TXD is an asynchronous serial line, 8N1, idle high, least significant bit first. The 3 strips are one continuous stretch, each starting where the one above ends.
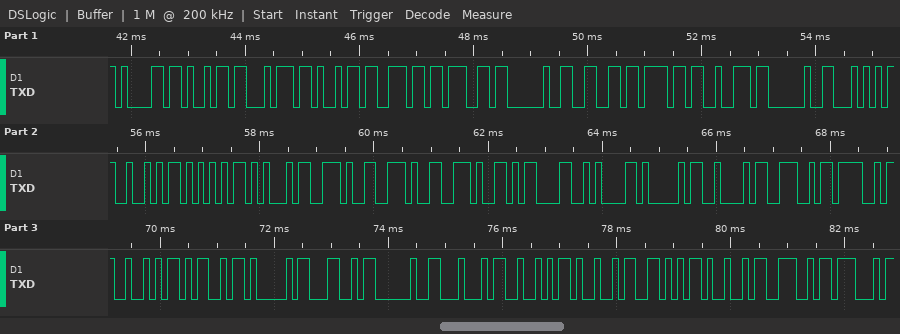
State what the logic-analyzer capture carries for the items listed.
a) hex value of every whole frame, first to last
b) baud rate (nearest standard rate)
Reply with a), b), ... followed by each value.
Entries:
a) 0x61 0x69 0x74 0x69 0x6E 0x67 0x20 0x66 0x6F 0x72 0x20 0x54 0x52 0x55 0x45 0x2E 0x2E 0x2E 0x0D 0x0A 0x41 0x42 0x4E 0x4F 0x52 0x4D 0x41 0x4C 0x20 0x44 0x52 0x49 0x56 0x49 0x4E 0x47
b) 9600 baud
